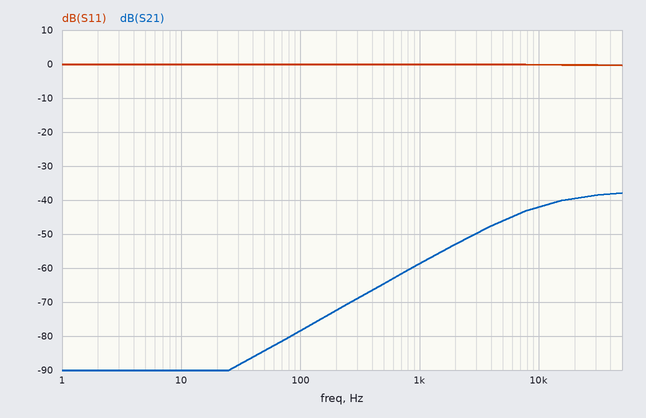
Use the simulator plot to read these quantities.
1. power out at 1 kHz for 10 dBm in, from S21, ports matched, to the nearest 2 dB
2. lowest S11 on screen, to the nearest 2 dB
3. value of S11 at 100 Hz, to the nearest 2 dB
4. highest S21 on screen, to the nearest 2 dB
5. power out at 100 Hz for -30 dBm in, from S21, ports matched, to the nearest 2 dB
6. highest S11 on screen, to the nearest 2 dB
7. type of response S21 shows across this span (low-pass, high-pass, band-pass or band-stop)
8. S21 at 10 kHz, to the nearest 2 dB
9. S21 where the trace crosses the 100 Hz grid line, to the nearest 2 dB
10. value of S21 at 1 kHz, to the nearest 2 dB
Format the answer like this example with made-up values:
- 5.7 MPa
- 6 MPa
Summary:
- -48 dBm
- 0 dB
- 0 dB
- -38 dB
- -108 dBm
- 0 dB
- high-pass
- -42 dB
- -78 dB
- -58 dB
